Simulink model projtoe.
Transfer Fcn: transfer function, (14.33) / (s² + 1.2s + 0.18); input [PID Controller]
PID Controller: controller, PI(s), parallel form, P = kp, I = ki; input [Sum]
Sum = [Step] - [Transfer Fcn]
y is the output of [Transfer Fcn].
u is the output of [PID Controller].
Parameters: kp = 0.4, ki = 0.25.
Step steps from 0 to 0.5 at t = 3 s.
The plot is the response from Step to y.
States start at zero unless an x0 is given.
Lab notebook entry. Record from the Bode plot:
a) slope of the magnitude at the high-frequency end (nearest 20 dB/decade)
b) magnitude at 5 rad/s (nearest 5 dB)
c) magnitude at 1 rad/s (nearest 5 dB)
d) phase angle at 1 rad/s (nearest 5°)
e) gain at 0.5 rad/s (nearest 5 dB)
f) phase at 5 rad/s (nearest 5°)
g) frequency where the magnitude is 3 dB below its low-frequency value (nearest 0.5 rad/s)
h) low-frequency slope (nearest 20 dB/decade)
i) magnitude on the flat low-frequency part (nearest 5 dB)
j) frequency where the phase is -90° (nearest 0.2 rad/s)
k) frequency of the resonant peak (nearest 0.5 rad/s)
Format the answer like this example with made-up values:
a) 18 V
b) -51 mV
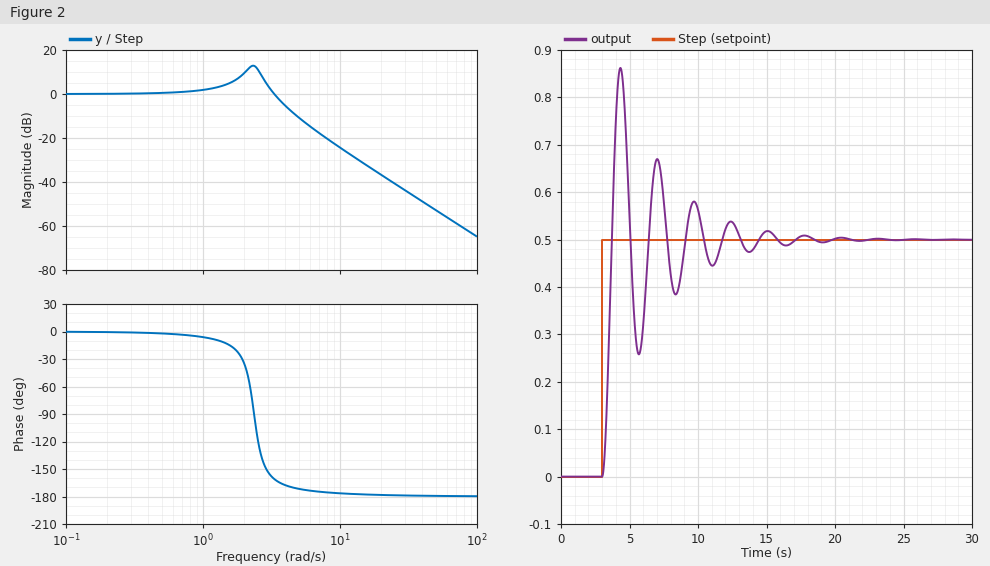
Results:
a) -40 dB/decade
b) -10 dB
c) 0 dB
d) -5°
e) 0 dB
f) -170°
g) 3.5 rad/s
h) 0 dB/decade
i) 0 dB
j) 2.4 rad/s
k) 2.5 rad/s
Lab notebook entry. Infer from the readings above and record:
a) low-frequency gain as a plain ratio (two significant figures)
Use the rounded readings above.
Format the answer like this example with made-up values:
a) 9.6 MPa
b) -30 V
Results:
a) 1.0
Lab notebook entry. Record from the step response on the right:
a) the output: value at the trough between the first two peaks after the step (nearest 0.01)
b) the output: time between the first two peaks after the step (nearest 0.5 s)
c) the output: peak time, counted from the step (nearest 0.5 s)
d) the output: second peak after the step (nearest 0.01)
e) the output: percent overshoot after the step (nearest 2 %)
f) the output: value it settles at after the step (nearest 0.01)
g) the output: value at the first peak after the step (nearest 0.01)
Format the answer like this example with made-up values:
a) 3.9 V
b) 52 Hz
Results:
a) 0.26
b) 2.5 s
c) 1.5 s
d) 0.67
e) 72 %
f) 0.50
g) 0.86
